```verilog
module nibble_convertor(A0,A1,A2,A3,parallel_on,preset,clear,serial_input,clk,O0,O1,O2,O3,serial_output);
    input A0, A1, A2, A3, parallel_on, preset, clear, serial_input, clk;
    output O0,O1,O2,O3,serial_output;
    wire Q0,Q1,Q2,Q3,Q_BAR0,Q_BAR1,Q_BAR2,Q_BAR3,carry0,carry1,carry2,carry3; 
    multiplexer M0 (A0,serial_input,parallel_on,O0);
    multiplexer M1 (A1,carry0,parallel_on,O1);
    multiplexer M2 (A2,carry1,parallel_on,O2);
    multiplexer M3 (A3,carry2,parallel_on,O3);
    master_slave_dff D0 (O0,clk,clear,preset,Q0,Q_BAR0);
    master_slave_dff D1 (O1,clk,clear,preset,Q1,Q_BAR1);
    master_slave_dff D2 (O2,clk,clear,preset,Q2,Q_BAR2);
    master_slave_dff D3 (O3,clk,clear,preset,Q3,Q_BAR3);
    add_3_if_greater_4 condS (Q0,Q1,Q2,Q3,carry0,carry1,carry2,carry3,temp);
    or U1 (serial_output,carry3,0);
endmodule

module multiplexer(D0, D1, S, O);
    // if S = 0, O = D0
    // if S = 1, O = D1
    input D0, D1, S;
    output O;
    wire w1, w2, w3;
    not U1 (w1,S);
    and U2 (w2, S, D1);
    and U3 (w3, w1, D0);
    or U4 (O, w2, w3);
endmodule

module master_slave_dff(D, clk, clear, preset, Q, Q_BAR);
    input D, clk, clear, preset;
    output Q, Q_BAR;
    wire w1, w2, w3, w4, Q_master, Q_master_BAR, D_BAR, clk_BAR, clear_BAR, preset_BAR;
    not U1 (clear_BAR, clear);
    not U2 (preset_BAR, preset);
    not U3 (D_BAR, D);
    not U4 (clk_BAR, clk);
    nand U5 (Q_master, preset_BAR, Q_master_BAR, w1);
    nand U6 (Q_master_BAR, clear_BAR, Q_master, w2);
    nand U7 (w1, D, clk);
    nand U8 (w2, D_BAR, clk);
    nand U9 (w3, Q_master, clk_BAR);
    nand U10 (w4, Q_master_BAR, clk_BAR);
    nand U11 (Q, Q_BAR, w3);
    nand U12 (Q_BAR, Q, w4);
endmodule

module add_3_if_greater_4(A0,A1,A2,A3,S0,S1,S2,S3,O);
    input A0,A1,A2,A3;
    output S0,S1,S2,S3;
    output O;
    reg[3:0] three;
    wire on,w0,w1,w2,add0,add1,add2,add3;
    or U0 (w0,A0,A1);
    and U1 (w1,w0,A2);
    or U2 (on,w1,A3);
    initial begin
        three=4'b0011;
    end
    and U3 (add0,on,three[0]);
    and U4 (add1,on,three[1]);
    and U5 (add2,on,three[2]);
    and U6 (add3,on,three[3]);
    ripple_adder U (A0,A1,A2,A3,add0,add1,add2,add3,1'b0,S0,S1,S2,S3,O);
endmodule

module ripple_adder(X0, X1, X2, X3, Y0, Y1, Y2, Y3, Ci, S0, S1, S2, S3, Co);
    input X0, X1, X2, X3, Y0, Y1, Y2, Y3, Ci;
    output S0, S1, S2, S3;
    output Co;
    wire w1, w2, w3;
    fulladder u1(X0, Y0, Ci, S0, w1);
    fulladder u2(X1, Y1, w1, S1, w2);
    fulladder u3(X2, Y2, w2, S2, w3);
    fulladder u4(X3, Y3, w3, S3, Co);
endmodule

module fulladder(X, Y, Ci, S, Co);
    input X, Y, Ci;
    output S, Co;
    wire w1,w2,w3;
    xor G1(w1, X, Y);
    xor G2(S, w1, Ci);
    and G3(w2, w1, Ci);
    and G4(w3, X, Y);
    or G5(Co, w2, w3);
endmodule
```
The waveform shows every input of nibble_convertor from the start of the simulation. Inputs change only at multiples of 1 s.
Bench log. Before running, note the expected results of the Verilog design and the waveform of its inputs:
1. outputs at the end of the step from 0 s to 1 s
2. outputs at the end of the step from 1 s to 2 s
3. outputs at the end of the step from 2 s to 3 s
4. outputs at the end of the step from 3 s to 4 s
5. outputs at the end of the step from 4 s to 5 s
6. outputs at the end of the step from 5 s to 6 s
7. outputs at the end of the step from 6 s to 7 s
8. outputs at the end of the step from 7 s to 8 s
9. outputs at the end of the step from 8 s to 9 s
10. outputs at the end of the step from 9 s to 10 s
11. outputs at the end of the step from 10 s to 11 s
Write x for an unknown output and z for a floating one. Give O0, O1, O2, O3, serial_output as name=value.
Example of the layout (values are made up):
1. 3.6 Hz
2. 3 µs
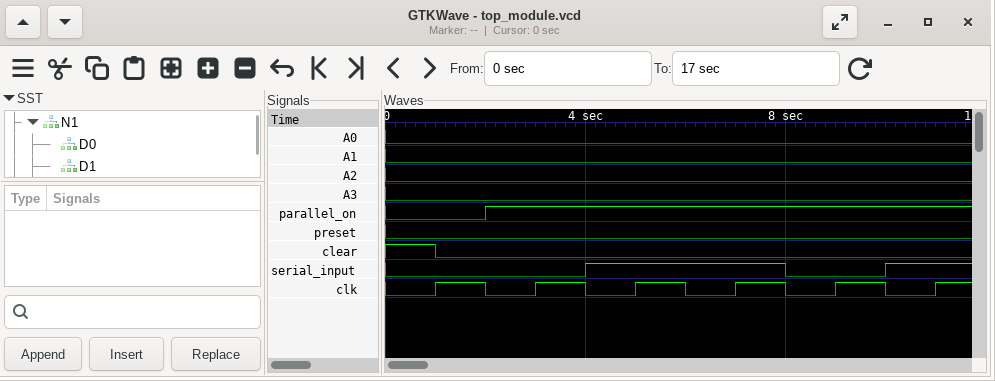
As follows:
1. O0=0, O1=0, O2=0, O3=0, serial_output=0
2. O0=0, O1=0, O2=0, O3=0, serial_output=0
3. O0=0, O1=0, O2=0, O3=0, serial_output=0
4. O0=0, O1=0, O2=0, O3=0, serial_output=0
5. O0=1, O1=0, O2=0, O3=0, serial_output=0
6. O0=1, O1=0, O2=0, O3=0, serial_output=0
7. O0=1, O1=1, O2=0, O3=0, serial_output=0
8. O0=1, O1=1, O2=0, O3=0, serial_output=0
9. O0=0, O1=1, O2=1, O3=0, serial_output=0
10. O0=0, O1=1, O2=1, O3=0, serial_output=0
11. O0=1, O1=1, O2=0, O3=0, serial_output=1
